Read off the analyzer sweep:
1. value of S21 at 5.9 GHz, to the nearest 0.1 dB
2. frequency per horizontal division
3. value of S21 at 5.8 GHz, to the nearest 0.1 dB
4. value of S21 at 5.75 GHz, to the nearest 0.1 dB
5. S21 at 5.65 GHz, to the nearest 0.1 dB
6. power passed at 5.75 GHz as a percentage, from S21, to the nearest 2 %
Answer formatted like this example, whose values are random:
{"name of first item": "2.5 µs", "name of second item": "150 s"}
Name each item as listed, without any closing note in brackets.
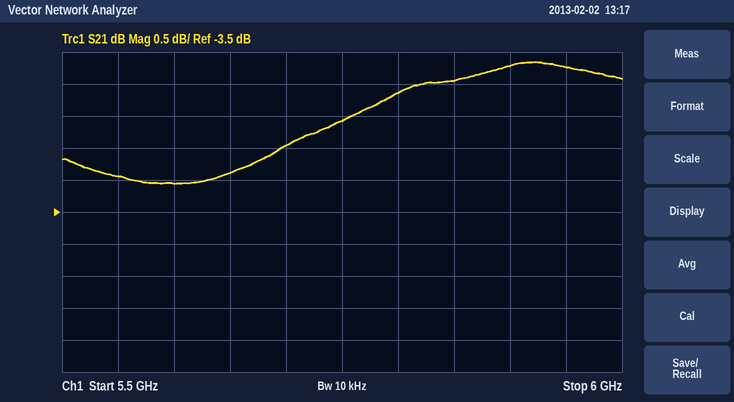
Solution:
{"value of S21 at 5.9 GHz, to the nearest 0.1 dB": "-1.2 dB", "frequency per horizontal division": "50 MHz", "value of S21 at 5.8 GHz, to the nearest 0.1 dB": "-1.6 dB", "value of S21 at 5.75 GHz, to the nearest 0.1 dB": "-2.1 dB", "S21 at 5.65 GHz, to the nearest 0.1 dB": "-2.9 dB", "power passed at 5.75 GHz as a percentage, from S21, to the nearest 2 %": "62 %"}
